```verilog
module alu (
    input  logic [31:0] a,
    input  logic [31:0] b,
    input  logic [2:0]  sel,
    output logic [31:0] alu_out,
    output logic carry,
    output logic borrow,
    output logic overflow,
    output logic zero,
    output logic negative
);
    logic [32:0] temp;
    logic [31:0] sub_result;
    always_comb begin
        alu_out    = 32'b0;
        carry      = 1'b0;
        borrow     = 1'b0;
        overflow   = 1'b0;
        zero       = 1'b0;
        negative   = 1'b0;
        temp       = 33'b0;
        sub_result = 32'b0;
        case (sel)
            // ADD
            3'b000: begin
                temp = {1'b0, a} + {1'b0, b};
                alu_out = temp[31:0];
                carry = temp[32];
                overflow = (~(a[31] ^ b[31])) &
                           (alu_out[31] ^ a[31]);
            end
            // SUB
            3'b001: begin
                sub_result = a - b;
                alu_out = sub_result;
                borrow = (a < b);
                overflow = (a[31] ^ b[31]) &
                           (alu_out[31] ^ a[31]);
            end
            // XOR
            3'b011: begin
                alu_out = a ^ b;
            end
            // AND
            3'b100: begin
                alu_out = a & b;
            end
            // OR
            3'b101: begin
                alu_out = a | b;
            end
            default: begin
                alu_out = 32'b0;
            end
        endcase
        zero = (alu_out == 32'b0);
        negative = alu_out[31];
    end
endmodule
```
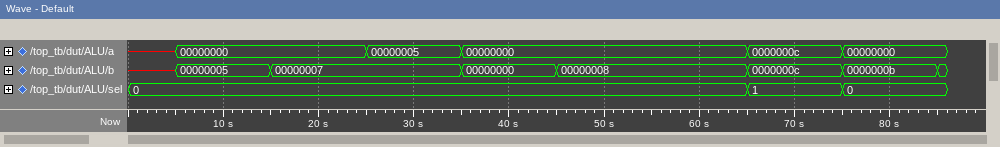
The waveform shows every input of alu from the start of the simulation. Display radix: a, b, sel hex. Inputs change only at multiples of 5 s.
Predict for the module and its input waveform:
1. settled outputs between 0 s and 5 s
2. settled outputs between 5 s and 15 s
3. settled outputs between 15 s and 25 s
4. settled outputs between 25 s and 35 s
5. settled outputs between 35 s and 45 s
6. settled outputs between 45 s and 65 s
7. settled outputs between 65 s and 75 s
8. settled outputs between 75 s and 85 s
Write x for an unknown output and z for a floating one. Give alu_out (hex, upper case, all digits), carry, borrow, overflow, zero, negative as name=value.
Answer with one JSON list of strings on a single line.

["alu_out=x, carry=x, borrow=0, overflow=x, zero=x, negative=x", "alu_out=00000005, carry=0, borrow=0, overflow=0, zero=0, negative=0", "alu_out=00000007, carry=0, borrow=0, overflow=0, zero=0, negative=0", "alu_out=0000000C, carry=0, borrow=0, overflow=0, zero=0, negative=0", "alu_out=00000000, carry=0, borrow=0, overflow=0, zero=1, negative=0", "alu_out=00000008, carry=0, borrow=0, overflow=0, zero=0, negative=0", "alu_out=00000000, carry=0, borrow=0, overflow=0, zero=1, negative=0", "alu_out=0000000B, carry=0, borrow=0, overflow=0, zero=0, negative=0"]
